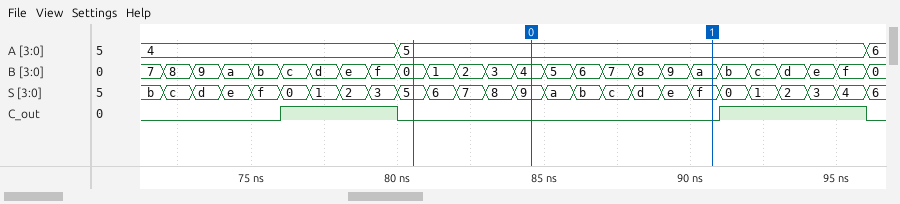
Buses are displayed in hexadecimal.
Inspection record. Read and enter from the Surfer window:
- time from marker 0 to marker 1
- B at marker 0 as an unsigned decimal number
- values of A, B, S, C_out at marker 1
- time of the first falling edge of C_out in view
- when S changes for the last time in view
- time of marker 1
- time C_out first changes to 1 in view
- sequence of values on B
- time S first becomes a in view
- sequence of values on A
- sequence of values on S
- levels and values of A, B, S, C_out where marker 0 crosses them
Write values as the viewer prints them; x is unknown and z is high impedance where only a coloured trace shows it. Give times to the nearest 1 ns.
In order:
6 ns
4
A=5, B=a, S=f, C_out=0
80 ns
96 ns
91 ns
76 ns
7, 8, 9, a, b, c, d, e, f, 0, 1, 2, 3, 4, 5, 6, 7, 8, 9, a, b, c, d, e, f, 0
85 ns
4, 5, 6
b, c, d, e, f, 0, 1, 2, 3, 5, 6, 7, 8, 9, a, b, c, d, e, f, 0, 1, 2, 3, 4, 6
A=5, B=4, S=9, C_out=0
